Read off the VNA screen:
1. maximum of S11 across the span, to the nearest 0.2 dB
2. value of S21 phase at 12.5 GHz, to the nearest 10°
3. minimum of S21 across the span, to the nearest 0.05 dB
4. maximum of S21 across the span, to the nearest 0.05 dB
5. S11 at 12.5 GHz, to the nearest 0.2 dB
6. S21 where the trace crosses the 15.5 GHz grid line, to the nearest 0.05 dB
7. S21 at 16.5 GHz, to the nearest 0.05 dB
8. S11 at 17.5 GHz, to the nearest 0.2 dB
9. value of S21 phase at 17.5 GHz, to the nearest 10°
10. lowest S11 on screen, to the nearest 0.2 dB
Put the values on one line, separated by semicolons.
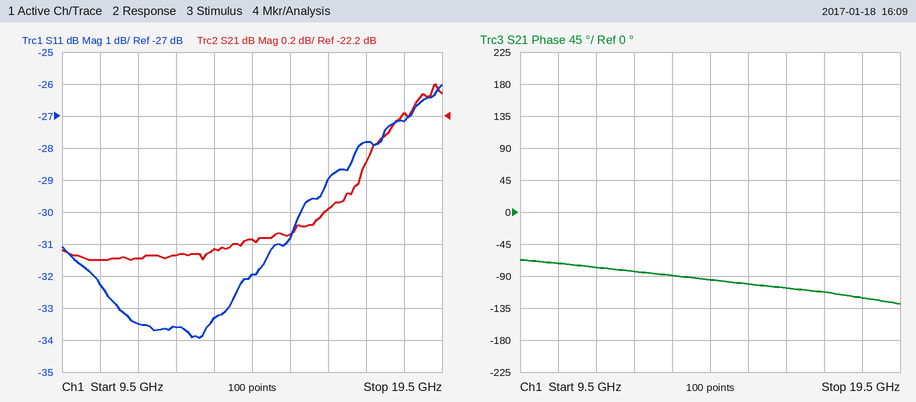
-26.0 dB; -80°; -23.10 dB; -22.00 dB; -33.6 dB; -22.95 dB; -22.80 dB; -27.8 dB; -110°; -34.0 dB
